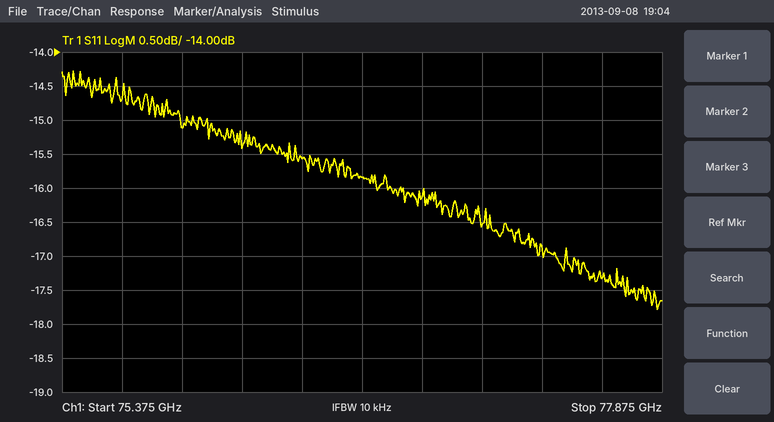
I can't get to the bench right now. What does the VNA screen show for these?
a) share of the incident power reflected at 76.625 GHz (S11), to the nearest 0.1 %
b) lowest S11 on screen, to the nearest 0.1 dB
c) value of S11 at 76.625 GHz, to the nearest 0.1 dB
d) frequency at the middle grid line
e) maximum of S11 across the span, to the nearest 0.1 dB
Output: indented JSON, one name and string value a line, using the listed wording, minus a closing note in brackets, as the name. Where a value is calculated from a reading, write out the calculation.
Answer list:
{
  "share of the incident power reflected at 76.625 GHz (S11), to the nearest 0.1 %": "10^(-15.8/10) ≈ 2.6 %",
  "lowest S11 on screen, to the nearest 0.1 dB": "-17.8 dB",
  "value of S11 at 76.625 GHz, to the nearest 0.1 dB": "-15.8 dB",
  "frequency at the middle grid line": "76.625 GHz",
  "maximum of S11 across the span, to the nearest 0.1 dB": "-14.3 dB"
}
